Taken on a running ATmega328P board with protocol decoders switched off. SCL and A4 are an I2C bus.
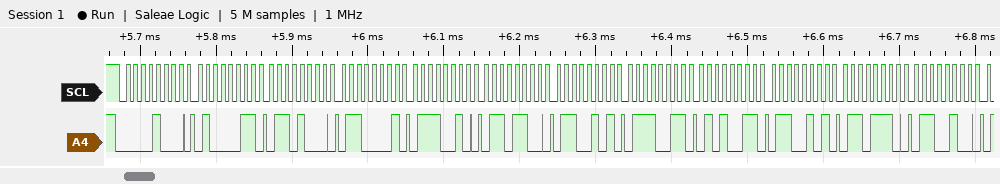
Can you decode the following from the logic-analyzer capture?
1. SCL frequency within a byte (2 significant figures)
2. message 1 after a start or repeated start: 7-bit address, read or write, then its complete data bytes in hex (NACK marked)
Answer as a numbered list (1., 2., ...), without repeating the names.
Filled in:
1. 100 kHz
2. 0x04 write: 43 68 61 72 6C 65 73 53 65 6E 64
